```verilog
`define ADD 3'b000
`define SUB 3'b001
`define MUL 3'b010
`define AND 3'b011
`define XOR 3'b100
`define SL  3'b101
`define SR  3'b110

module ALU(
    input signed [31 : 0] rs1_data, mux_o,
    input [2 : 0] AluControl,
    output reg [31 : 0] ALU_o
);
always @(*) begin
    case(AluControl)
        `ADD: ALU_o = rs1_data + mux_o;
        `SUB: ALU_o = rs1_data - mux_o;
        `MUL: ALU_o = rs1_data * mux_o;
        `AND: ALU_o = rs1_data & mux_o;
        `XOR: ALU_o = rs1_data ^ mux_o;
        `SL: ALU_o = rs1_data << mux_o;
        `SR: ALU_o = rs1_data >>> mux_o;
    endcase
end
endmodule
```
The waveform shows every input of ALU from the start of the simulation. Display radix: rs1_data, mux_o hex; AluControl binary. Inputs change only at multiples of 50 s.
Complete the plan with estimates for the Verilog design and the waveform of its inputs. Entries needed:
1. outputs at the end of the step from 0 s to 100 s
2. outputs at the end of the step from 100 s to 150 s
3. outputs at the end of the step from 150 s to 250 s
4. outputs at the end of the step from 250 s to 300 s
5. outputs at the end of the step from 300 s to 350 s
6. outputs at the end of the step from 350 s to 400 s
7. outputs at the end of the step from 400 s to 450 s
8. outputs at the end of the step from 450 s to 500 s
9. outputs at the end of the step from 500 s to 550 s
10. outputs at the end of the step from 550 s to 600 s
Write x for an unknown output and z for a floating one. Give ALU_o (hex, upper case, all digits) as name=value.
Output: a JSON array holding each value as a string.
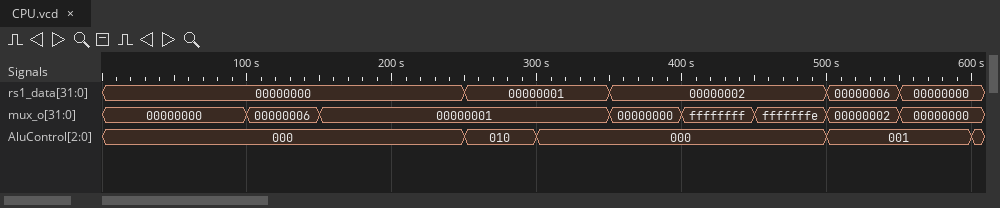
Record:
["ALU_o=00000000", "ALU_o=00000006", "ALU_o=00000001", "ALU_o=00000001", "ALU_o=00000002", "ALU_o=00000002", "ALU_o=00000001", "ALU_o=00000000", "ALU_o=00000004", "ALU_o=00000000"]
